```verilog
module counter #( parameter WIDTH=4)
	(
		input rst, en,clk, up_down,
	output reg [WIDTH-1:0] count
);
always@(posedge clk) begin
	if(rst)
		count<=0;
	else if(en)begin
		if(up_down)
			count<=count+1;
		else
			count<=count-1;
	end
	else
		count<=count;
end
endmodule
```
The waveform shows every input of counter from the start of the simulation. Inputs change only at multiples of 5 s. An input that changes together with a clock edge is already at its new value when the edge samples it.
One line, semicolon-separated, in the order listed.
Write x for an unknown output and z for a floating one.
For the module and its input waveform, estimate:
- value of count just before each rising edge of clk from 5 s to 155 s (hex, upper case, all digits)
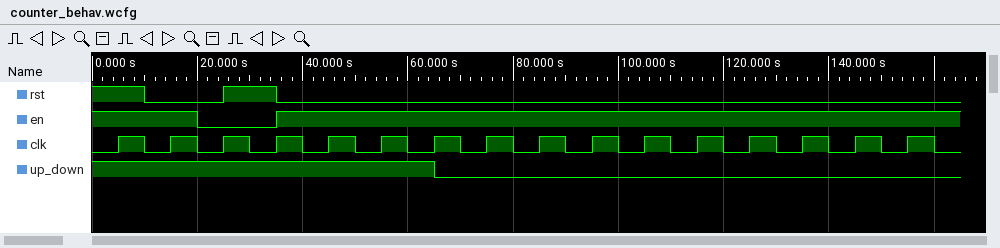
x, 0, 1, 0, 1, 2, 3, 2, 1, 0, F, E, D, C, B, A
